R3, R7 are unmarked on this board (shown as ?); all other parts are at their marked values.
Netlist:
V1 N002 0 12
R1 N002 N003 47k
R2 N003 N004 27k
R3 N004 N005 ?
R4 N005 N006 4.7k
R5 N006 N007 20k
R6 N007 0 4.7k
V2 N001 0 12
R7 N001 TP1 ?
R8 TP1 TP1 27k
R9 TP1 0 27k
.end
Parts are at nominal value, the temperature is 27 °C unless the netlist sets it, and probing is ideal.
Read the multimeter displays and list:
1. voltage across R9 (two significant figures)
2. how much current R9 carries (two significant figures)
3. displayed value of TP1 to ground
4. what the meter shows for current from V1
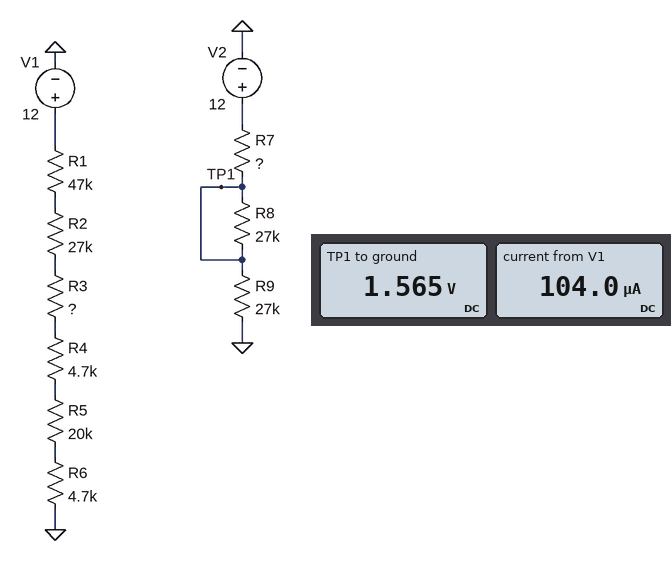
1.6 V
58 µA
1.565 V
104.0 µA
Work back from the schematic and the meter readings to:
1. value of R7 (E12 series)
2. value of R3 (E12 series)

180 kΩ
12 kΩ
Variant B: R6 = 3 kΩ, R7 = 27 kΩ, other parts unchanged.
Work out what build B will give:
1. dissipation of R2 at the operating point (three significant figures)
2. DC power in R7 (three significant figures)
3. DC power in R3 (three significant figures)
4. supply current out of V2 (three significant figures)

301 µW
1.33 mW
134 µW
222 µA
